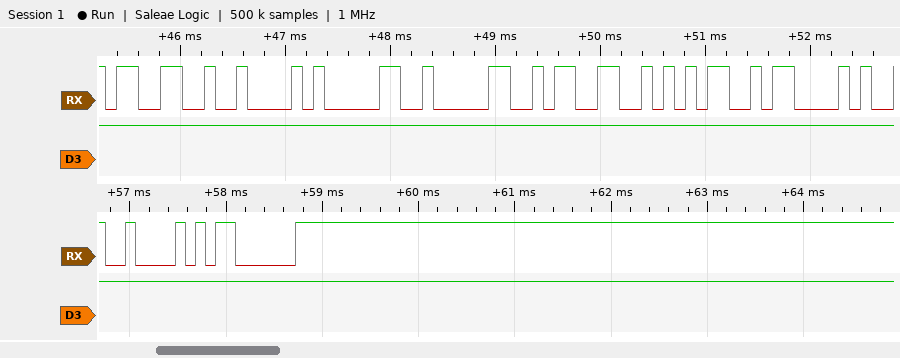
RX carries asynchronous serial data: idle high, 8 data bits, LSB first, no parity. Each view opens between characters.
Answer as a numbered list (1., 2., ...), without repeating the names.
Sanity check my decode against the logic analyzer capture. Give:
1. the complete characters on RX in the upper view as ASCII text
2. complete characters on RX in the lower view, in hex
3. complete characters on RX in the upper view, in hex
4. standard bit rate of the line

1. "3B0035C"
2. 42, 03
3. 33, 42, 30, 30, 33, 35, 43
4. 9600 baud
